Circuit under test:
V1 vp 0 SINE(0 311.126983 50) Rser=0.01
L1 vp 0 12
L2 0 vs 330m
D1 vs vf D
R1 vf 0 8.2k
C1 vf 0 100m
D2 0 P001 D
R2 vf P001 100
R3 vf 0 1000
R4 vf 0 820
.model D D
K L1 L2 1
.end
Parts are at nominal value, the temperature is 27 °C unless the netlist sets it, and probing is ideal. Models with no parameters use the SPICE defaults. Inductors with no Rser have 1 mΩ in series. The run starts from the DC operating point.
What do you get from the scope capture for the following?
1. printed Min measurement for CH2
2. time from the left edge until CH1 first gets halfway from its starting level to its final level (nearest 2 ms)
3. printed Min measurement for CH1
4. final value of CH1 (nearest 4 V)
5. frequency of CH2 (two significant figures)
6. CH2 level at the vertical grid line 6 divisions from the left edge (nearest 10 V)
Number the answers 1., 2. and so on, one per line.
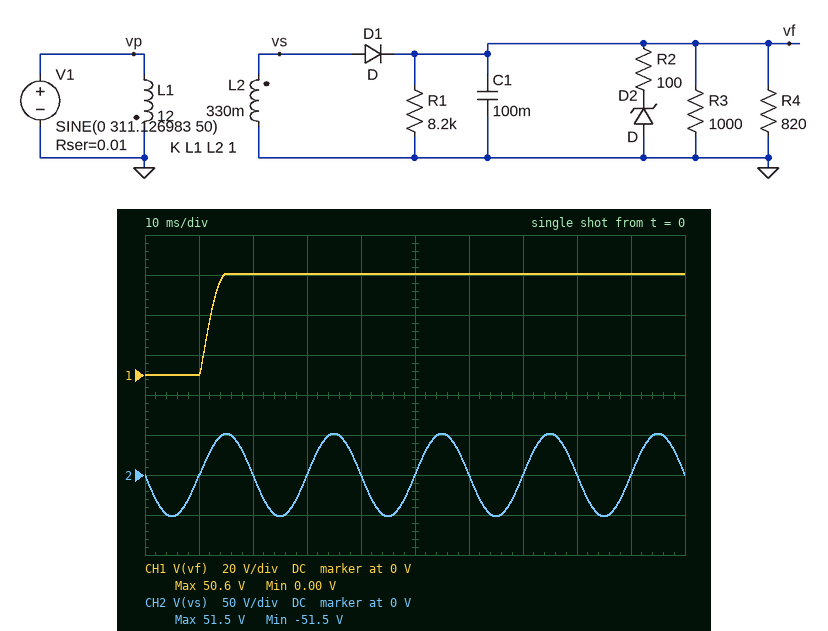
1. -51.5 V
2. 12 ms
3. 0.00 V
4. 52 V
5. 50 Hz
6. 0 V
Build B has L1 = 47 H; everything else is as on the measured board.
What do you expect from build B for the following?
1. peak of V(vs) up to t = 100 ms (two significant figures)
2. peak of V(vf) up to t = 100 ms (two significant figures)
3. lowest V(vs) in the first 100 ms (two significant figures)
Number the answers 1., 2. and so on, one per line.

1. 26 V
2. 25 V
3. -26 V
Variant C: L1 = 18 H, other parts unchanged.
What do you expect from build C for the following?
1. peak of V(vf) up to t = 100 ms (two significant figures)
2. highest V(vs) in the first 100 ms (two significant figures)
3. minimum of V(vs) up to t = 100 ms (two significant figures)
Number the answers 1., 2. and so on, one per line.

1. 41 V
2. 42 V
3. -42 V
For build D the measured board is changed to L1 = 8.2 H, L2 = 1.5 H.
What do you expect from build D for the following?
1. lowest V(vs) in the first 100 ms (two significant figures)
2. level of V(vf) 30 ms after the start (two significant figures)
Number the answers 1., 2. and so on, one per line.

1. -130 V
2. 130 V
